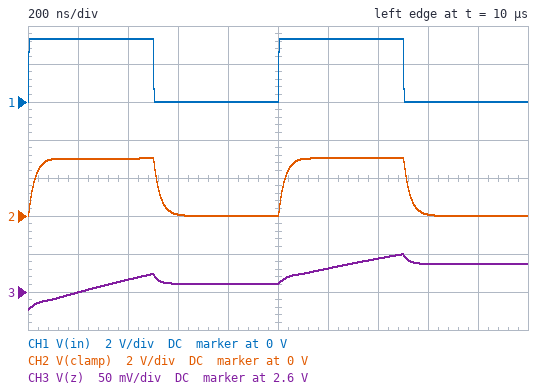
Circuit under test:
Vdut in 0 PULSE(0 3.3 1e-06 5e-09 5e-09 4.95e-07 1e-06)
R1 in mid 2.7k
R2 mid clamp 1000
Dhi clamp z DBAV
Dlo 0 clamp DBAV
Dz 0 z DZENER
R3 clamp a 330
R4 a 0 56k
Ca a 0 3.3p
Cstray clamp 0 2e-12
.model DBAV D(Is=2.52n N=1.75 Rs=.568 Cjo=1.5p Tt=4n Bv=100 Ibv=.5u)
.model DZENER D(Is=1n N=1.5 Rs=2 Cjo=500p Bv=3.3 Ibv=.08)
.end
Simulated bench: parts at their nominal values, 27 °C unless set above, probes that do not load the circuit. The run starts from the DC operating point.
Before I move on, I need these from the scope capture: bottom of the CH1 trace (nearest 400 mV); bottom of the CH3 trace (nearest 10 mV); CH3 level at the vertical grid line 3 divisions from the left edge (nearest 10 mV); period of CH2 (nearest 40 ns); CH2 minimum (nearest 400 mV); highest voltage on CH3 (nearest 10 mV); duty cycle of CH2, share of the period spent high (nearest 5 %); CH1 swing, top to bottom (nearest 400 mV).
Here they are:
0 V
2.58 V
2.61 V
1.00 µs
0 V
2.65 V
50 %
3.2 V
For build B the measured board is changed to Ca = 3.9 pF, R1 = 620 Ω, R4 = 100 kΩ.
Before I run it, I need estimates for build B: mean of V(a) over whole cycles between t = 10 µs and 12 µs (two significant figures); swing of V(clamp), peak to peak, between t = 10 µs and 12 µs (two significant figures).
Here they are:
1.6 V
3.2 V
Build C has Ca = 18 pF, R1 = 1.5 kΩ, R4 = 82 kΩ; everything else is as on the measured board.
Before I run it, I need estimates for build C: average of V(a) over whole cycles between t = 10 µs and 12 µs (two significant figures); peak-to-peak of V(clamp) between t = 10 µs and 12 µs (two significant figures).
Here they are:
1.6 V
3.2 V
